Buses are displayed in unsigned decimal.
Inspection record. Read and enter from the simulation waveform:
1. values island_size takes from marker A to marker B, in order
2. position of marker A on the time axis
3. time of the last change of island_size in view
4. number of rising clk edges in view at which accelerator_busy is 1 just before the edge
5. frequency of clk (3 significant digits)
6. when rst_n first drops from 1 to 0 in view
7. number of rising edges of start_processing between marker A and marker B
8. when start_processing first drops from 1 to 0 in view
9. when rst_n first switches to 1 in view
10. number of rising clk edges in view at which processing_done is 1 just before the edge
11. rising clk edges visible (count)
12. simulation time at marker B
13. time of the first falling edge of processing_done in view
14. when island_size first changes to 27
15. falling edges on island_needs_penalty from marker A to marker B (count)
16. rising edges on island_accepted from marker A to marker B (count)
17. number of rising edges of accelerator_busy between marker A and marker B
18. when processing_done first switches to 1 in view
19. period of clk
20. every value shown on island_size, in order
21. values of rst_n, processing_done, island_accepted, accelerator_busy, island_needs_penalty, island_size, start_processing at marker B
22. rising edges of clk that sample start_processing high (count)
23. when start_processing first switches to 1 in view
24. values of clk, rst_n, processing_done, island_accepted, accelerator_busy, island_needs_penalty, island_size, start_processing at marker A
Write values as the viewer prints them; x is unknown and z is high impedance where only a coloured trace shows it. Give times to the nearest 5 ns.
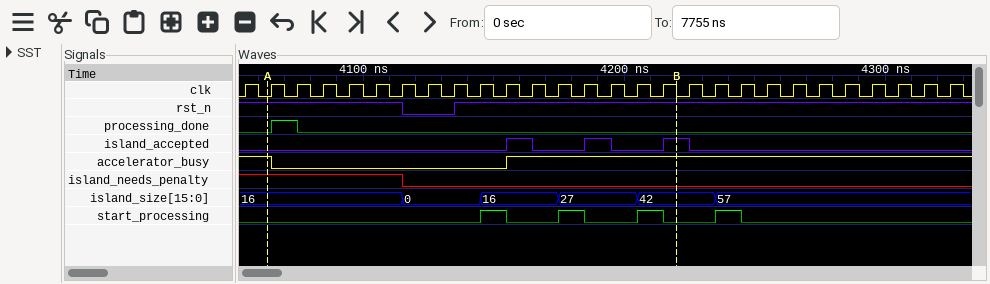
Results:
16, 0, 16, 27, 42
4065 ns
4235 ns
19
100 MHz
4115 ns
3
4155 ns
4135 ns
1
28
4220 ns
4075 ns
4175 ns
1
3
1
4065 ns
10 ns
16, 0, 16, 27, 42, 57
rst_n=1, processing_done=0, island_accepted=1, accelerator_busy=1, island_needs_penalty=0, island_size=42, start_processing=0
4
4145 ns
clk=0, rst_n=1, processing_done=0, island_accepted=0, accelerator_busy=1, island_needs_penalty=1, island_size=16, start_processing=0
